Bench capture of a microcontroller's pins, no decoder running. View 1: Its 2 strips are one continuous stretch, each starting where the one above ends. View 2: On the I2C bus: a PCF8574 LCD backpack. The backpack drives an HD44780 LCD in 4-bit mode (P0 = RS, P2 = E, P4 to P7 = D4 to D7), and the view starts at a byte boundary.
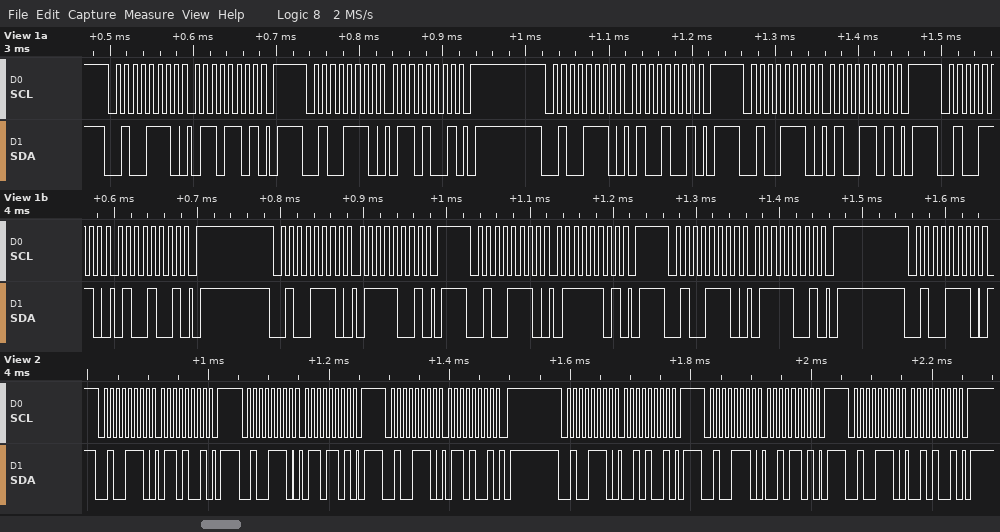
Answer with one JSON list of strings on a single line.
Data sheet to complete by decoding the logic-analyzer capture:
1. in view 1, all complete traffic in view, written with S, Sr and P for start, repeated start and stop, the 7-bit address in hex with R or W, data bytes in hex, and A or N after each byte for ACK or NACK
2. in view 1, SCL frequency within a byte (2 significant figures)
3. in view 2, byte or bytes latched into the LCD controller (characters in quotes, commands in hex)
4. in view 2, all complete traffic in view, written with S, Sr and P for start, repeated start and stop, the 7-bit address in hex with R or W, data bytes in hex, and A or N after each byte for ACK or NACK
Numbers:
["S 27W A 6D A P S 27W A 69 A P S 27W A 49 A P S 27W A 4D A P S 27W A 49 A P S 27W A 79 A P S 27W A 7D A P S 27W A 79 A P S 27W A", "100 kHz", "'b'", "S 27W A 69 A P S 27W A 6D A P S 27W A 69 A P S 27W A 29 A P S 27W A 2D A P S 27W A 29 A P"]
